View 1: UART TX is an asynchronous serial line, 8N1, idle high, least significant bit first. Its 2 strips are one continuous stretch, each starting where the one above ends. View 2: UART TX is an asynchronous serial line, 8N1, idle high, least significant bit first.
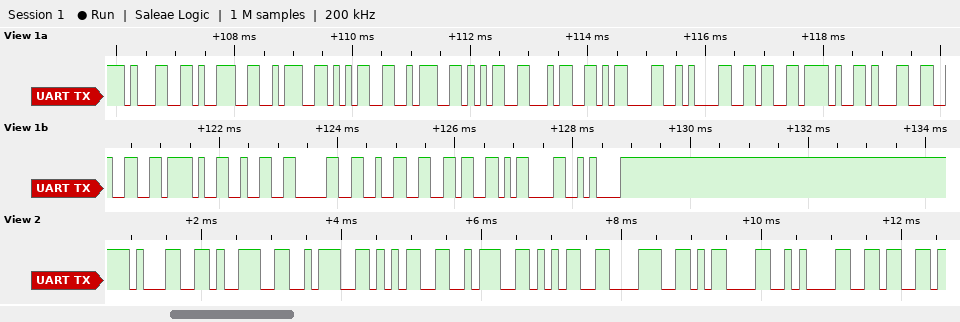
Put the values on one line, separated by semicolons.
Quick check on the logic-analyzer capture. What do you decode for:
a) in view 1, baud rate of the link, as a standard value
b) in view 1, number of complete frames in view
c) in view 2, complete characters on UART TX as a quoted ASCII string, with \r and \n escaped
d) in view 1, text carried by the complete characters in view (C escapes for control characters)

9600 baud; 20; "19:5:58\r\n6"; "19:5:54\r\n6/12/2026\r\n"
